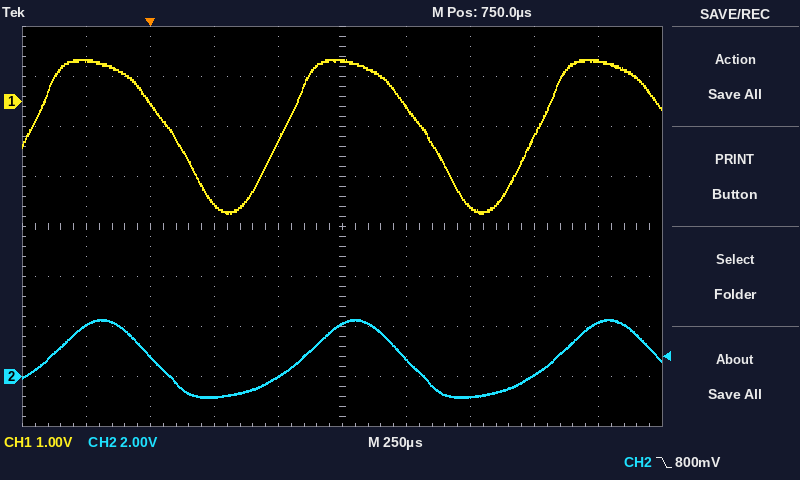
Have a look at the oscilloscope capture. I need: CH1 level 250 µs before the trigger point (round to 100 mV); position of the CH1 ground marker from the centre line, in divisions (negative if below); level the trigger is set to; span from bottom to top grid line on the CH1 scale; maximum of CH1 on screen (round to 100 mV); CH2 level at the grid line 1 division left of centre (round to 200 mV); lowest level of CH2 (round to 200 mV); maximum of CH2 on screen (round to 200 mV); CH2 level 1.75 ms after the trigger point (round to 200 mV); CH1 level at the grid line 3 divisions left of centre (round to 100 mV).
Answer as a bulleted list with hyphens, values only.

- 800 mV
- +2.5 div
- 800 mV
- 8 V
- 800 mV
- 0.0 V
- -800 mV
- 2.2 V
- 2.2 V
- 0.0 V
